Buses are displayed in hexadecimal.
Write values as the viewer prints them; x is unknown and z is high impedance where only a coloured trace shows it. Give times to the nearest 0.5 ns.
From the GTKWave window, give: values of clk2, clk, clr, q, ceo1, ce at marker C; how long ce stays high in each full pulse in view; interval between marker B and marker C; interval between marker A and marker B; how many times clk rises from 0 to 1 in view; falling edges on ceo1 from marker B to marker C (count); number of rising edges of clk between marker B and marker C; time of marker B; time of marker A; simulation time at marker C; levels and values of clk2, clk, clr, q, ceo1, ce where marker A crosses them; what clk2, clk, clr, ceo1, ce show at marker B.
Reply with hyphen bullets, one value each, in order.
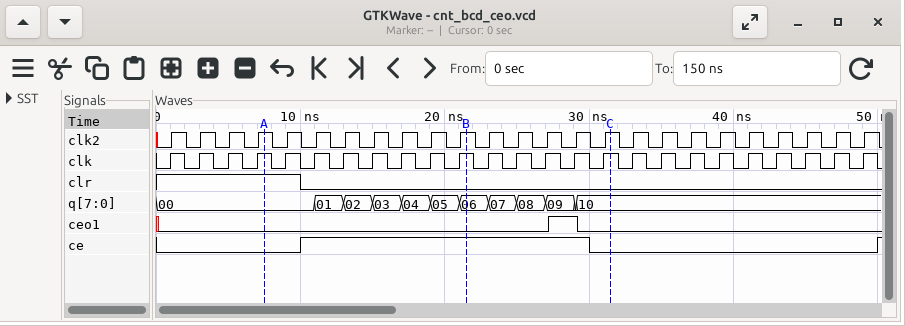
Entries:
- clk2=1, clk=1, clr=0, q=10, ceo1=0, ce=0
- 20 ns
- 10 ns
- 14 ns
- 25
- 1
- 5
- 21.5 ns
- 7.5 ns
- 31.5 ns
- clk2=1, clk=1, clr=1, q=00, ceo1=0, ce=0
- clk2=1, clk=1, clr=0, ceo1=0, ce=1
